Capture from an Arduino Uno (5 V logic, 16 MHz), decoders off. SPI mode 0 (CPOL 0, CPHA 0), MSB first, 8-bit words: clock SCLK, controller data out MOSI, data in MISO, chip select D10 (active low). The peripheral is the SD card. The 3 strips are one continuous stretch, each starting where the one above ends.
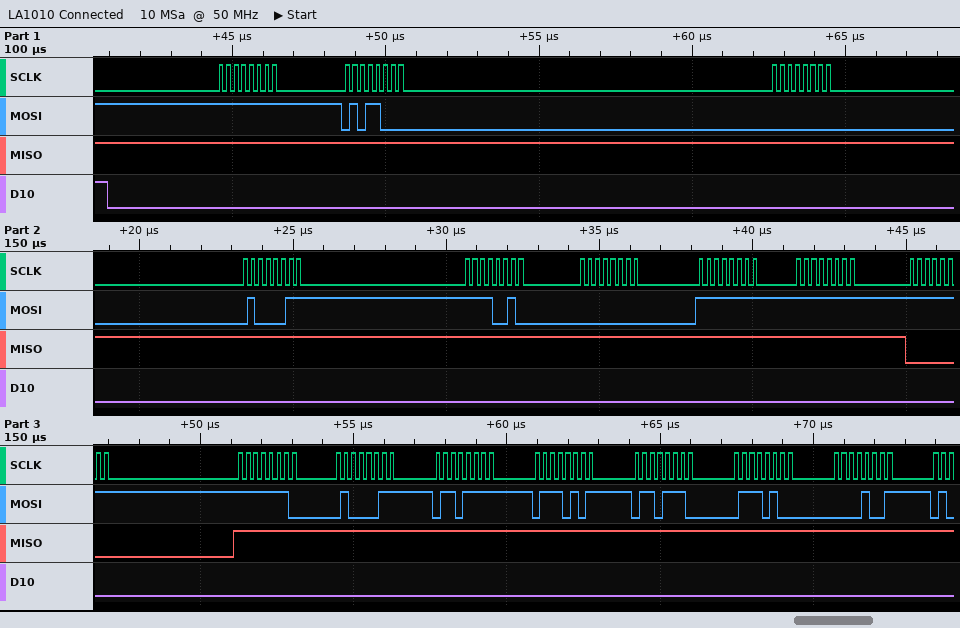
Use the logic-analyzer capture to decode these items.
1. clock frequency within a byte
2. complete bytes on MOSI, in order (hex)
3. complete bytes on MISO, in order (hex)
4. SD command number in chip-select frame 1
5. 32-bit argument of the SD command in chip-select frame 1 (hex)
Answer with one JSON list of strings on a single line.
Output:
["4 MHz", "FF 58 00 43 F2 00 FF FF FF FE 43 6F 75 6E 74 09", "FF FF FF FF FF FF FF FF 00 FF FF FF FF FF FF FF", "CMD24", "0x0043F200"]
